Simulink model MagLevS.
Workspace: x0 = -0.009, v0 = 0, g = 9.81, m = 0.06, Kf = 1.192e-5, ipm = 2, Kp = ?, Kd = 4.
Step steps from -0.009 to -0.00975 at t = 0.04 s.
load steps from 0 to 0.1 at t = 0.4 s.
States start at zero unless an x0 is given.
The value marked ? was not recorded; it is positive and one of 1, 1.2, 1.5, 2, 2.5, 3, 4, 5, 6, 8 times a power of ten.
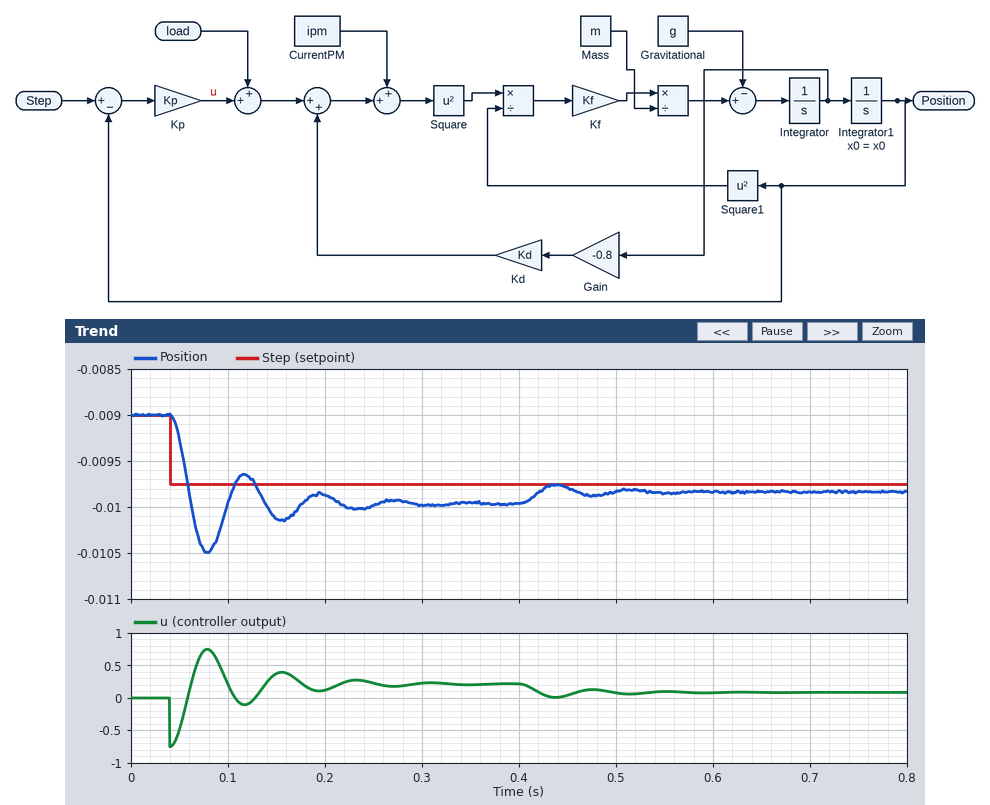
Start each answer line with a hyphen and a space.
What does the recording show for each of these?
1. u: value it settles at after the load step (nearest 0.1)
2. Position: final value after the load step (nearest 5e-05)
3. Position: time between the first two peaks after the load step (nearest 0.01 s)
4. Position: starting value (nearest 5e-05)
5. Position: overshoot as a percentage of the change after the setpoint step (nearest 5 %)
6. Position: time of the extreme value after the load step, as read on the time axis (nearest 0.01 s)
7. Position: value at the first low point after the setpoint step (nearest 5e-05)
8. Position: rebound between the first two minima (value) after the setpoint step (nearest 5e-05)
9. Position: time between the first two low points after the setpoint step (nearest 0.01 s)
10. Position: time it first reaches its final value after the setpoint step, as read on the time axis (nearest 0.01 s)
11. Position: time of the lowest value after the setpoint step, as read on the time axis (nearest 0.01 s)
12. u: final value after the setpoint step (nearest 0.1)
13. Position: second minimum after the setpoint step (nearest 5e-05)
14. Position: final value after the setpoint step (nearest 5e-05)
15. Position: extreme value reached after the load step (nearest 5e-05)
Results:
- 0.1
- -0.00985
- 0.08 s
- -0.00900
- 55 %
- 0.44 s
- -0.01050
- -0.00965
- 0.08 s
- 0.06 s
- 0.08 s
- 0.2
- -0.01015
- -0.00995
- -0.00975
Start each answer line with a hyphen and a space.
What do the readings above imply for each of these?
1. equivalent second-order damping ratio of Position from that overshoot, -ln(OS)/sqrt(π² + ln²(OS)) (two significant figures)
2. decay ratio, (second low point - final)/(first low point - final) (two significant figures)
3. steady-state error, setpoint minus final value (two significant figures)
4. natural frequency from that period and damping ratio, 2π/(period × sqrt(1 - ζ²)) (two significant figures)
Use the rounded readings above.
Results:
- 0.19
- 0.36
- 0.00020
- 80 rad/s
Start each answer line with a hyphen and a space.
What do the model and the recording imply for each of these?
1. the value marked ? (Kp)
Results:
- 1000
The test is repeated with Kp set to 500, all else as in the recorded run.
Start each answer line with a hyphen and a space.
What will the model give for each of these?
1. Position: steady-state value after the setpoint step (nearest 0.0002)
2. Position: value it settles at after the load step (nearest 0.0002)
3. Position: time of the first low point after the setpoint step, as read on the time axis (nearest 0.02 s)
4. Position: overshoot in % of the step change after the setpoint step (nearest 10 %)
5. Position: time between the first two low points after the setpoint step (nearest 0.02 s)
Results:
- -0.0104
- -0.0100
- 0.10 s
- 40 %
- 0.14 s
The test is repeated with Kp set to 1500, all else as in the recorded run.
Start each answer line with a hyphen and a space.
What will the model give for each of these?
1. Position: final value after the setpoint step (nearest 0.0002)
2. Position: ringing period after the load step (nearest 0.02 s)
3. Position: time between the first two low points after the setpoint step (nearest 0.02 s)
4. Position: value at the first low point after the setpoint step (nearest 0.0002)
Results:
- -0.0098
- 0.06 s
- 0.06 s
- -0.0104
